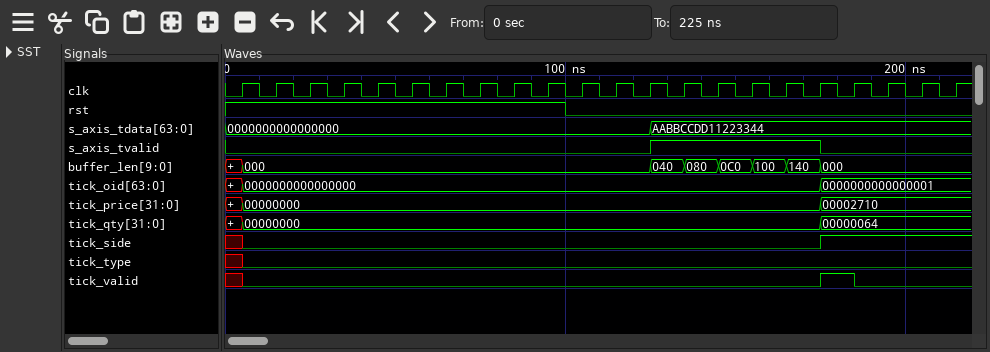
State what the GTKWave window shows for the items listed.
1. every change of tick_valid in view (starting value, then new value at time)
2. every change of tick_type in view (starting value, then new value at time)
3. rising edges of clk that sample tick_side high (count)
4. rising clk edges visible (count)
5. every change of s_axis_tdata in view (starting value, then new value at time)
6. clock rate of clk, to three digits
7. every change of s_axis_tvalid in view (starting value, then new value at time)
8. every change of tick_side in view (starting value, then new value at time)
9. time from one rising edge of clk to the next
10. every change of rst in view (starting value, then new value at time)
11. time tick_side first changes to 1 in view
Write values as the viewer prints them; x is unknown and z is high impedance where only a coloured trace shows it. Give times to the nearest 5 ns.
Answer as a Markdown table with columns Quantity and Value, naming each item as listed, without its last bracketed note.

| Quantity | Value |
|---|---|
| every change of tick_valid in view | x, 0 at 5 ns, 1 at 175 ns, 0 at 185 ns |
| every change of tick_type in view | x, 0 at 5 ns |
| rising edges of clk that sample tick_side high | 4 |
| rising clk edges visible | 22 |
| every change of s_axis_tdata in view | 0000000000000000, AABBCCDD11223344 at 125 ns |
| clock rate of clk, to three digits | 100 MHz |
| every change of s_axis_tvalid in view | 0, 1 at 125 ns, 0 at 175 ns |
| every change of tick_side in view | x, 0 at 5 ns, 1 at 175 ns |
| time from one rising edge of clk to the next | 10 ns |
| every change of rst in view | 1, 0 at 100 ns |
| time tick_side first changes to 1 in view | 175 ns |
